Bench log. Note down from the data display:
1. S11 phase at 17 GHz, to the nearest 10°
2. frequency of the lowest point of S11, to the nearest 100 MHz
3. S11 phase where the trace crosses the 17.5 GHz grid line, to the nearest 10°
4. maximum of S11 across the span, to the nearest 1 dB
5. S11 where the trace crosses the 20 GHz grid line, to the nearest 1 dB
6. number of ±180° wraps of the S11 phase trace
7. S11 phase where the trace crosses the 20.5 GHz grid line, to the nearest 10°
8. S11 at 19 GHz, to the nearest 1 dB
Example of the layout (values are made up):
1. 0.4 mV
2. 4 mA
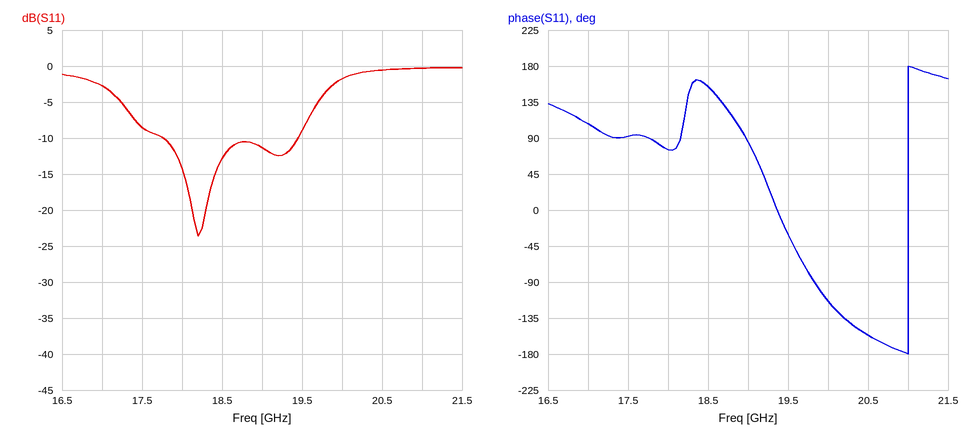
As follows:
1. 110°
2. 18.2 GHz
3. 90°
4. 0 dB
5. -2 dB
6. 1
7. -160°
8. -11 dB
